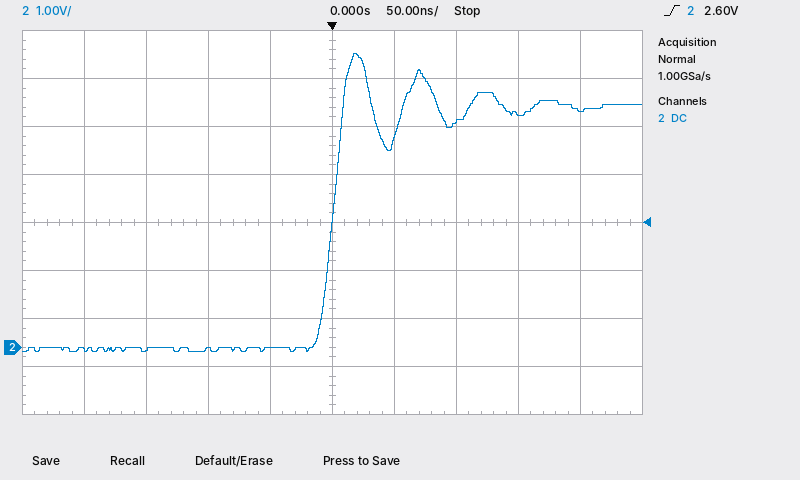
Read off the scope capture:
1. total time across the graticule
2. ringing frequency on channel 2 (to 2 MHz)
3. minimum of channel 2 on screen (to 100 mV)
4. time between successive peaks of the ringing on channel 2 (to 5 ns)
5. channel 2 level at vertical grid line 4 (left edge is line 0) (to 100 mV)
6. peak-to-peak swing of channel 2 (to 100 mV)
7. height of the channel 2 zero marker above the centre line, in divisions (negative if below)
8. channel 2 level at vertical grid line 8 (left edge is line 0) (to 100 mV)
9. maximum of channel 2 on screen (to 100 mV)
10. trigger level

500 ns
20 MHz
-100 mV
50 ns
0.0 V
6.2 V
-2.6 div
4.9 V
6.1 V
2.60 V
